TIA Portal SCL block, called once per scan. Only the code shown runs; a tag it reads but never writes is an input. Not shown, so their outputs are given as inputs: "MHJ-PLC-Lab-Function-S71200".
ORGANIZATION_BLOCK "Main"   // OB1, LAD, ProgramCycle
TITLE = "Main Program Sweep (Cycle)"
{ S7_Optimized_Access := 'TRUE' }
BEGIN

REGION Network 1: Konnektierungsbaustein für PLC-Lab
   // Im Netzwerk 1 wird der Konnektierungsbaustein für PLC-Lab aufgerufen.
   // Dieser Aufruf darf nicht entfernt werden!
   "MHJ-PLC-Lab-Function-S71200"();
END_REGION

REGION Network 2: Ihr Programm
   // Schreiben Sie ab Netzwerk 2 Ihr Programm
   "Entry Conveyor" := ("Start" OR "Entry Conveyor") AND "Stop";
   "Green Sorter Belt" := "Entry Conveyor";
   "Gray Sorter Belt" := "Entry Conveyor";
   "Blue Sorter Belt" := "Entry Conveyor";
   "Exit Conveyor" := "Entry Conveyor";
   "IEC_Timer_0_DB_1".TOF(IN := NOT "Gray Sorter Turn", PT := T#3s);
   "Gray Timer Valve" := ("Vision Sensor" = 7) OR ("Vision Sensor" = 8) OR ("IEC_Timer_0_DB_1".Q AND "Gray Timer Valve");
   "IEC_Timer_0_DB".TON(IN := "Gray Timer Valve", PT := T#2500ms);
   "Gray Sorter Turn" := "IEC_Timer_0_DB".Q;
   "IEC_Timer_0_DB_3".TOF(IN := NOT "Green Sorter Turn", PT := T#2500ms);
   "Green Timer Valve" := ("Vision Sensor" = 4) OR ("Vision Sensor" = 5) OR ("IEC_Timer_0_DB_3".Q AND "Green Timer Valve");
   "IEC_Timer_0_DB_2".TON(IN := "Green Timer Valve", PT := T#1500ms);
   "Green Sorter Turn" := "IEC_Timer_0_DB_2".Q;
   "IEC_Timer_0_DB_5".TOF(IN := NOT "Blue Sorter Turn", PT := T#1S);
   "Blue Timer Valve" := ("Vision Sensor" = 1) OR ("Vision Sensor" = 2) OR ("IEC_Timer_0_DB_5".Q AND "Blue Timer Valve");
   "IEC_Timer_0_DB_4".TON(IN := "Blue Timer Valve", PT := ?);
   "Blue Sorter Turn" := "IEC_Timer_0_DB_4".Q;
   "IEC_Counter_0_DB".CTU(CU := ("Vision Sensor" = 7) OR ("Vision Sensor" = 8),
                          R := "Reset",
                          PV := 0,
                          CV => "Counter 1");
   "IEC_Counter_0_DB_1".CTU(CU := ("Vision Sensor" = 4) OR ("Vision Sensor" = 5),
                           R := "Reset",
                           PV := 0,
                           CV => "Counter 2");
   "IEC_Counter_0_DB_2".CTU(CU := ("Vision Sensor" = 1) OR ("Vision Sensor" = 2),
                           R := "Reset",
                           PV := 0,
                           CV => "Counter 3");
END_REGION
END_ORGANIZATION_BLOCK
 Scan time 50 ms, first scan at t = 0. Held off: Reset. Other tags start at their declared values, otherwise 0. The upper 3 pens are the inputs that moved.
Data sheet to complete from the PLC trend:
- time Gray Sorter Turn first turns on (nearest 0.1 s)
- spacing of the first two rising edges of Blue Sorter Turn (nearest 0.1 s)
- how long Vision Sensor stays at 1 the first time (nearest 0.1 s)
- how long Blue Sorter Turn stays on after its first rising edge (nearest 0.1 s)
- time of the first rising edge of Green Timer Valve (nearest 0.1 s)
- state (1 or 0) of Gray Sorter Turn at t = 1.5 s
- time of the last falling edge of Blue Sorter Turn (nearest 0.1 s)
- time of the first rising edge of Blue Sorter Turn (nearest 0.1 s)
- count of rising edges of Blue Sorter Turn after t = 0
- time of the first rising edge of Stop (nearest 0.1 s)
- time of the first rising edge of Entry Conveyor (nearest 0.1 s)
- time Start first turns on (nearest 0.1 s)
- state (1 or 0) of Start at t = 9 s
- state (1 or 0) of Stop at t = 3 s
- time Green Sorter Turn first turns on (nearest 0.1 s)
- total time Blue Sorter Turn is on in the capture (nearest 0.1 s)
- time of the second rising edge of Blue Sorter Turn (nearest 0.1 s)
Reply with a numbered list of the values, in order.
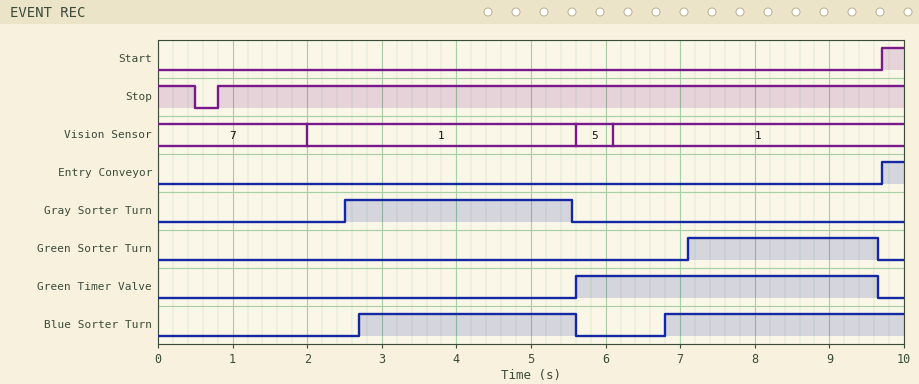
1. 2.5 s
2. 4.1 s
3. 3.6 s
4. 2.9 s
5. 5.6 s
6. 0
7. 5.6 s
8. 2.7 s
9. 2
10. 0.8 s
11. 9.7 s
12. 9.7 s
13. 0
14. 1
15. 7.1 s
16. 6.1 s
17. 6.8 s
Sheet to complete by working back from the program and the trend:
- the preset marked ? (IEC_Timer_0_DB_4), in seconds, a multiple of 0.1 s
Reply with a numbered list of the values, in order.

1. 0.7 s
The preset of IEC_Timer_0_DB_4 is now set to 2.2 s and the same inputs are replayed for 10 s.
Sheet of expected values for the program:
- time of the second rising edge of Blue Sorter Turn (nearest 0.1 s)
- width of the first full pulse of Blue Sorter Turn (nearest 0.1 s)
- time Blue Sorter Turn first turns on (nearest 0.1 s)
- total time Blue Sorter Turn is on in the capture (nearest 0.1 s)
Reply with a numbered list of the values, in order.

1. 8.3 s
2. 1.4 s
3. 4.2 s
4. 3.1 s
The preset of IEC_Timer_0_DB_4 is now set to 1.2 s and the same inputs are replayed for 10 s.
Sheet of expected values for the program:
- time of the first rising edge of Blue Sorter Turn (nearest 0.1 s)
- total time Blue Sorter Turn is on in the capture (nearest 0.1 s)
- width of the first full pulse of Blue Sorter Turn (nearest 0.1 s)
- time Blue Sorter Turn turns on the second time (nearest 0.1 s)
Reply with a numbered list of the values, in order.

1. 3.2 s
2. 5.1 s
3. 2.4 s
4. 7.3 s
